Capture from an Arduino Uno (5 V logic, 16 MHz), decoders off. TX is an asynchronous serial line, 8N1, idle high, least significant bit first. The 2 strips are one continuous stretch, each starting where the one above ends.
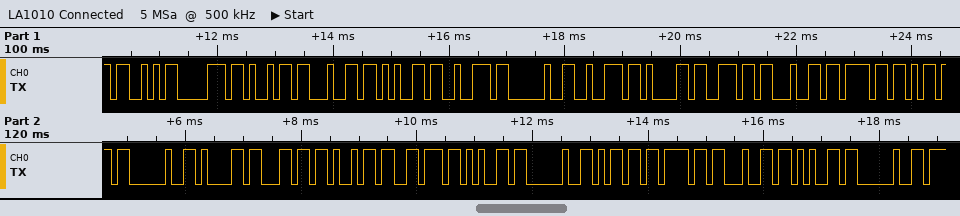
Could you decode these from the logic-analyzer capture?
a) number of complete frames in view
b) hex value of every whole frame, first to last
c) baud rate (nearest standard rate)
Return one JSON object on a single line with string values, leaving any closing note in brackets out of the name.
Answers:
{"number of complete frames in view": "25", "hex value of every whole frame, first to last": "53 70 69 64 65 72 20 72 61 6E 64 6F 6D 20 61 6C 69 76 65 20 6D 6F 64 65 20", "baud rate": "9600 baud"}
